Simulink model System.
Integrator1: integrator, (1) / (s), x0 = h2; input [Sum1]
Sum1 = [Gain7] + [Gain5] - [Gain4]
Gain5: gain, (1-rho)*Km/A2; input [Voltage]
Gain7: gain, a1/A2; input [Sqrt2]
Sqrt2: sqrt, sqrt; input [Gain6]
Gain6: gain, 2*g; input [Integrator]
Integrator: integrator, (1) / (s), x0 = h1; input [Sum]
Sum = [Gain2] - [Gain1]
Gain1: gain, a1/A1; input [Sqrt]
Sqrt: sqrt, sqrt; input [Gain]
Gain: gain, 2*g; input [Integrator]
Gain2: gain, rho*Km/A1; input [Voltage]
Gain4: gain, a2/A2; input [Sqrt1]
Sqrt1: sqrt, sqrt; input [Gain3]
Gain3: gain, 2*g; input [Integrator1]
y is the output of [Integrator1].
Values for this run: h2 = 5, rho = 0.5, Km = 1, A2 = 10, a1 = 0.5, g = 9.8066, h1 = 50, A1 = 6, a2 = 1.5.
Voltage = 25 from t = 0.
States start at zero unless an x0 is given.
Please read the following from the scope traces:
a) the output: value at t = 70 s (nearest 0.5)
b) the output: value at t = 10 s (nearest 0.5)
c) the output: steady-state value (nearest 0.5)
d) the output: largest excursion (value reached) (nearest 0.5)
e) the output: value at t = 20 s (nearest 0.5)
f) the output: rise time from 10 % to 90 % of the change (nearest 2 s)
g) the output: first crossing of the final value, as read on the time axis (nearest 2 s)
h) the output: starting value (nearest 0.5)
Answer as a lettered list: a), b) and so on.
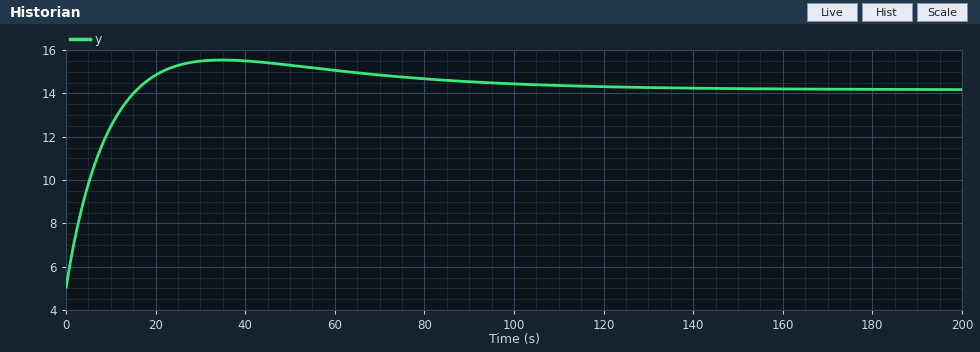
a) 15.0
b) 12.5
c) 14.0
d) 15.5
e) 15.0
f) 12 s
g) 16 s
h) 5.0
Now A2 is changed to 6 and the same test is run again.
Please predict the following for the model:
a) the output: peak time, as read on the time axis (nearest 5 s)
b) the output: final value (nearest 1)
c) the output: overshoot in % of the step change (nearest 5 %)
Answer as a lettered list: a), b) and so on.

a) 25 s
b) 14
c) 20 %
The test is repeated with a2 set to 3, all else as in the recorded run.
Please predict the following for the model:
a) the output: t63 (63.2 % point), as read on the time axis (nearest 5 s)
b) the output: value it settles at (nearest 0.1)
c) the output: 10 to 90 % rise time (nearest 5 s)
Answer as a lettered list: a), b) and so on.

a) 25 s
b) 3.5
c) 65 s
